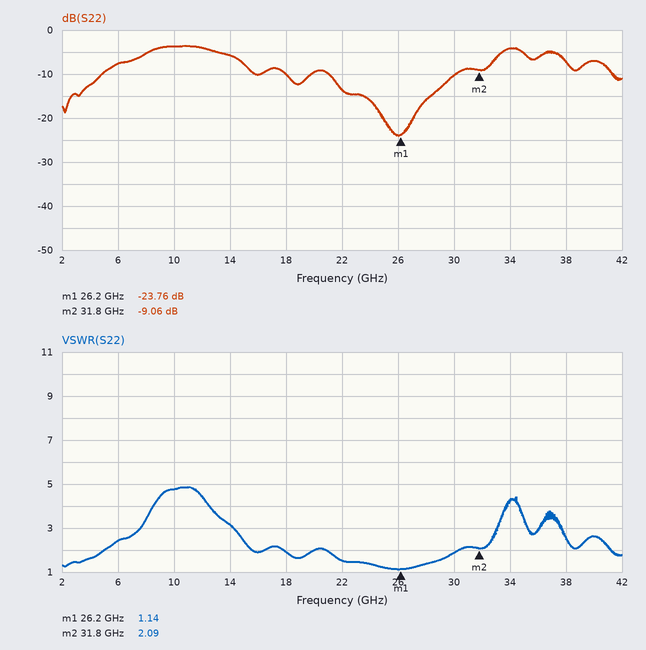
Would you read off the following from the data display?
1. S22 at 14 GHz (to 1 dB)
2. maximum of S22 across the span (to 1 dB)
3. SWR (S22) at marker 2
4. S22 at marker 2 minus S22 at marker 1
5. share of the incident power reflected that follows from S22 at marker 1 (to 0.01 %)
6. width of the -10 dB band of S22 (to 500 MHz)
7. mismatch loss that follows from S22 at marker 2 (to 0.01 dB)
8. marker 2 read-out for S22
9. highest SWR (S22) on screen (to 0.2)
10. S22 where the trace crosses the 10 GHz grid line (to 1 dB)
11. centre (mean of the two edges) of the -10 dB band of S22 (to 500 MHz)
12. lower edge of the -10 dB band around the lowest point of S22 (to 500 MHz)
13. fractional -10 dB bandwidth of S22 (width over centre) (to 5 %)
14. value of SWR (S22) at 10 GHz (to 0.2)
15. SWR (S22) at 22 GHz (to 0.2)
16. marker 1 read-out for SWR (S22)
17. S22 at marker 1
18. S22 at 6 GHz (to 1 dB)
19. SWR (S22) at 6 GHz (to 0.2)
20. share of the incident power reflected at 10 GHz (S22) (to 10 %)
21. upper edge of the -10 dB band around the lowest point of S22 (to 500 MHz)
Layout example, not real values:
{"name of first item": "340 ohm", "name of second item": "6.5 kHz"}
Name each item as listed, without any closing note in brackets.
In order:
{"S22 at 14 GHz": "-6 dB", "maximum of S22 across the span": "-4 dB", "SWR (S22) at marker 2": "2.09", "S22 at marker 2 minus S22 at marker 1": "14.70 dB", "share of the incident power reflected that follows from S22 at marker 1": "0.42 %", "width of the -10 dB band of S22": "9.0 GHz", "mismatch loss that follows from S22 at marker 2": "0.58 dB", "marker 2 read-out for S22": "-9.06 dB", "highest SWR (S22) on screen": "4.8", "S22 where the trace crosses the 10 GHz grid line": "-4 dB", "centre (mean of the two edges) of the -10 dB band of S22": "25.5 GHz", "lower edge of the -10 dB band around the lowest point of S22": "21.0 GHz", "fractional -10 dB bandwidth of S22 (width over centre)": "35 %", "value of SWR (S22) at 10 GHz": "4.8", "SWR (S22) at 22 GHz": "1.6", "marker 1 read-out for SWR": "1.14", "S22 at marker 1": "-23.76 dB", "S22 at 6 GHz": "-8 dB", "SWR (S22) at 6 GHz": "2.4", "share of the incident power reflected at 10 GHz (S22)": "40 %", "upper edge of the -10 dB band around the lowest point of S22": "30.0 GHz"}
